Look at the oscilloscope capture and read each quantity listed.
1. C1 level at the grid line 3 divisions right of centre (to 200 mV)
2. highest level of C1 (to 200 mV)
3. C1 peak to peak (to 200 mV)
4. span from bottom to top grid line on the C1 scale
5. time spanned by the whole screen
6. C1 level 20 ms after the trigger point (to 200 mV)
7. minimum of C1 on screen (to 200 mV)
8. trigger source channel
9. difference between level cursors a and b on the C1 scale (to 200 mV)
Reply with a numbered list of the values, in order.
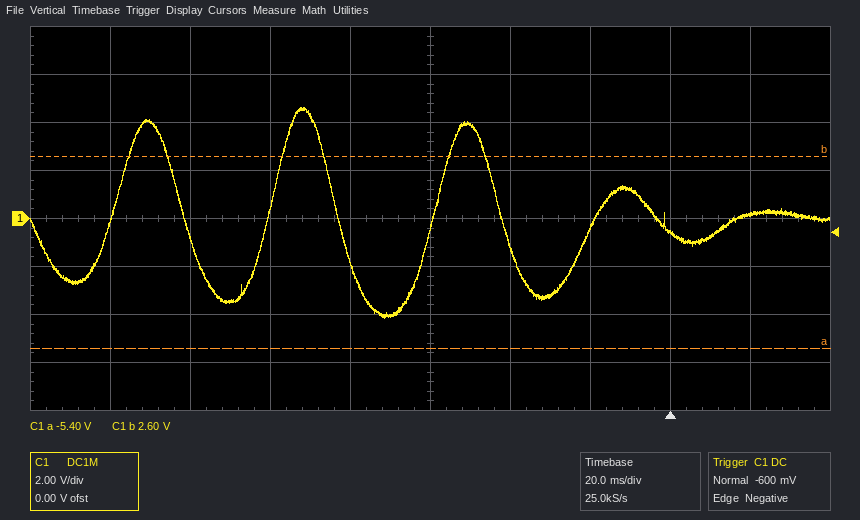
1. -600 mV
2. 4.6 V
3. 8.8 V
4. 16 V
5. 200 ms
6. 200 mV
7. -4.2 V
8. C1
9. 8.0 V
